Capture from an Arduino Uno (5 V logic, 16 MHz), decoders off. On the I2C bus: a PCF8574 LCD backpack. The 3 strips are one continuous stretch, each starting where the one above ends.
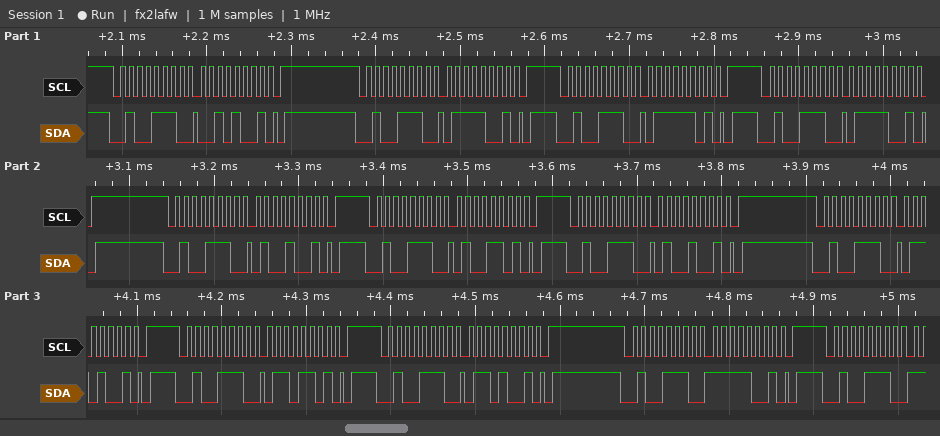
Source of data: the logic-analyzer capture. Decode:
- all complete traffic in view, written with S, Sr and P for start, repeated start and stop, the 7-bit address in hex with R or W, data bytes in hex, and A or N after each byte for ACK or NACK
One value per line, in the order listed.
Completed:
S 27W A 29 A P S 27W A 79 A P S 27W A 7D A P S 27W A 79 A P S 27W A 49 A P S 27W A 4D A P S 27W A 49 A P S 27W A 69 A P S 27W A 6D A P S 27W A 69 A P S 27W A F9 A P S 27W A
